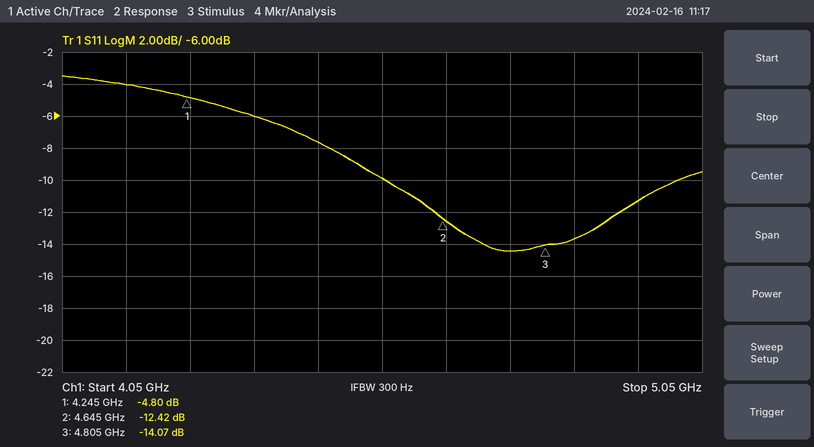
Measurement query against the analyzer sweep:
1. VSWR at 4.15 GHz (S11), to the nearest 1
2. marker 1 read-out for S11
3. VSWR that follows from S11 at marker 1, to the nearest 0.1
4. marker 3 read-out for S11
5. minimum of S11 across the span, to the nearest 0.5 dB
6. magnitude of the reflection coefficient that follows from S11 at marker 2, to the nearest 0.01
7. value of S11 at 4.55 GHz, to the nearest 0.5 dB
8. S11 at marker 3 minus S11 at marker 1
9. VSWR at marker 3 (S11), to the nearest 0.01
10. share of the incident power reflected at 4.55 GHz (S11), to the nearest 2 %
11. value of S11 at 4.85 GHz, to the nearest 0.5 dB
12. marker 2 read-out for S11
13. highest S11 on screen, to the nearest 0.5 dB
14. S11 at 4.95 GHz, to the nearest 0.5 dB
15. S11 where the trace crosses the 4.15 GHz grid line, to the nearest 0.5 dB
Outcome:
4
-4.80 dB
3.7
-14.07 dB
-14.5 dB
0.24
-10.0 dB
-9.27 dB
1.49
10 %
-13.5 dB
-12.42 dB
-3.5 dB
-11.5 dB
-4.0 dB
